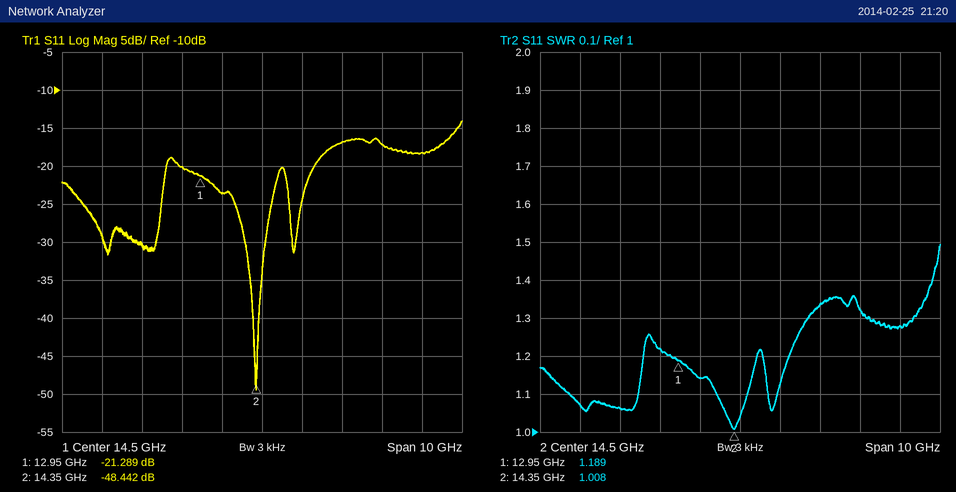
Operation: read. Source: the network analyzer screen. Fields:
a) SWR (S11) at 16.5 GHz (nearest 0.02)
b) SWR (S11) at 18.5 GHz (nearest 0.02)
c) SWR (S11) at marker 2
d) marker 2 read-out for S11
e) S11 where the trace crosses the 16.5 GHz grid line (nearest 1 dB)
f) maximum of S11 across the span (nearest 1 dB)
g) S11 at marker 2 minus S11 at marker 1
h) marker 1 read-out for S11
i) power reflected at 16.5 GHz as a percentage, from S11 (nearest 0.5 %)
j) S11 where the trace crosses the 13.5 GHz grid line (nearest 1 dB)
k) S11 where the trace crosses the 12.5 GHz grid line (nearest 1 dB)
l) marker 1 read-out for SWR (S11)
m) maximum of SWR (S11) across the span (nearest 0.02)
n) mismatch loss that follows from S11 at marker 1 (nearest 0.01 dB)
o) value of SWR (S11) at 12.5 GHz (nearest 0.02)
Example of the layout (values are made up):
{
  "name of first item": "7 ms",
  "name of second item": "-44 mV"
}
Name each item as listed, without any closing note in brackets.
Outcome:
{
  "SWR (S11) at 16.5 GHz": "1.34",
  "SWR (S11) at 18.5 GHz": "1.28",
  "SWR (S11) at marker 2": "1.008",
  "marker 2 read-out for S11": "-48.442 dB",
  "S11 where the trace crosses the 16.5 GHz grid line": "-17 dB",
  "maximum of S11 across the span": "-14 dB",
  "S11 at marker 2 minus S11 at marker 1": "-27.153 dB",
  "marker 1 read-out for S11": "-21.289 dB",
  "power reflected at 16.5 GHz as a percentage, from S11": "2.0 %",
  "S11 where the trace crosses the 13.5 GHz grid line": "-24 dB",
  "S11 where the trace crosses the 12.5 GHz grid line": "-20 dB",
  "marker 1 read-out for SWR": "1.189",
  "maximum of SWR (S11) across the span": "1.50",
  "mismatch loss that follows from S11 at marker 1": "0.03 dB",
  "value of SWR (S11) at 12.5 GHz": "1.22"
}
